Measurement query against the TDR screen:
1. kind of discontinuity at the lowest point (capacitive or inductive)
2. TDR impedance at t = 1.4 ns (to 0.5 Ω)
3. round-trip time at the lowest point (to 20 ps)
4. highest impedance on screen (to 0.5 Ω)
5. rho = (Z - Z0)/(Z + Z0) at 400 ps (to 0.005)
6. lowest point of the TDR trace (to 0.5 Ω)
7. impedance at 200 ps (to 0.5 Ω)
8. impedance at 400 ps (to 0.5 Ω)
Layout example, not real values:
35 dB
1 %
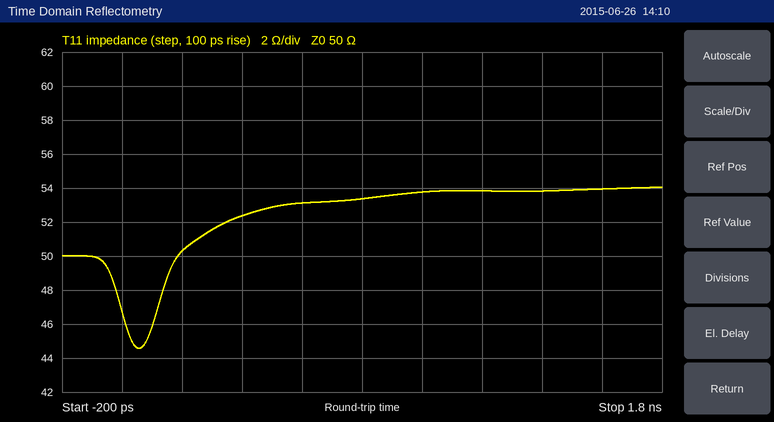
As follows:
capacitive
54.0 Ω
60 ps
54.0 Ω
+0.025
44.5 Ω
50.5 Ω
52.5 Ω
